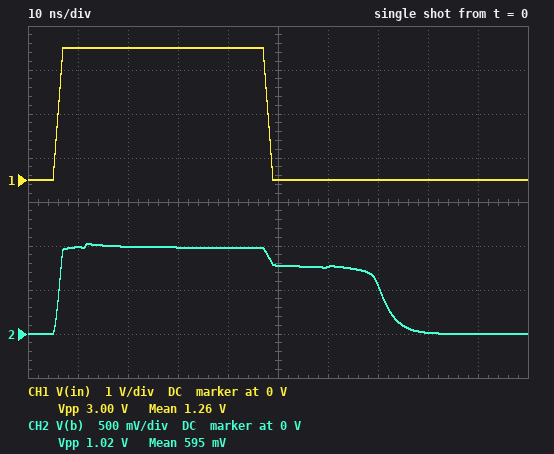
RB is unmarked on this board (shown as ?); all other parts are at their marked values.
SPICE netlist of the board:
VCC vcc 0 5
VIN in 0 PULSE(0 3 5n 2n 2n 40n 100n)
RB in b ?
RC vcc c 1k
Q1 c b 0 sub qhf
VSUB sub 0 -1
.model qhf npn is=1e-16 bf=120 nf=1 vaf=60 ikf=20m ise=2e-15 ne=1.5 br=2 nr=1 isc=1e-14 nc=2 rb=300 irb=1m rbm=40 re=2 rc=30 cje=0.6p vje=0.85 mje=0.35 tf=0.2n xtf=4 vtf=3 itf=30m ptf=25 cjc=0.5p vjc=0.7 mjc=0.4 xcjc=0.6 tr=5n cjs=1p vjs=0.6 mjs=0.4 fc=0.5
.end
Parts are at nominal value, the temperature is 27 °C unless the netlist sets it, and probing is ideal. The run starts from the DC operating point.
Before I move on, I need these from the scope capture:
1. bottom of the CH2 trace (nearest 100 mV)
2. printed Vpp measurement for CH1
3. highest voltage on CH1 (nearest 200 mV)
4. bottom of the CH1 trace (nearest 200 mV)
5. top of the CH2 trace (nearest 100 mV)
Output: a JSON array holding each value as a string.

["0 V", "3.00 V", "3.0 V", "0 V", "1.0 V"]
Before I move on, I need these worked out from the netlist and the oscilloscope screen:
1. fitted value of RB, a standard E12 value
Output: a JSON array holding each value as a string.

["2.7 kΩ"]
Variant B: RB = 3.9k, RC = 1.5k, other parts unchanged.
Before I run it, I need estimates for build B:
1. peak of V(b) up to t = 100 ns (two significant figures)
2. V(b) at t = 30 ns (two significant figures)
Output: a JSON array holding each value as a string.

["960 mV", "930 mV"]
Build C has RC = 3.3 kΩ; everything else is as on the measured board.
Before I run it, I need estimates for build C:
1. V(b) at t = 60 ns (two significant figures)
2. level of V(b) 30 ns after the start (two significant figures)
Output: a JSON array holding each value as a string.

["710 mV", "960 mV"]
